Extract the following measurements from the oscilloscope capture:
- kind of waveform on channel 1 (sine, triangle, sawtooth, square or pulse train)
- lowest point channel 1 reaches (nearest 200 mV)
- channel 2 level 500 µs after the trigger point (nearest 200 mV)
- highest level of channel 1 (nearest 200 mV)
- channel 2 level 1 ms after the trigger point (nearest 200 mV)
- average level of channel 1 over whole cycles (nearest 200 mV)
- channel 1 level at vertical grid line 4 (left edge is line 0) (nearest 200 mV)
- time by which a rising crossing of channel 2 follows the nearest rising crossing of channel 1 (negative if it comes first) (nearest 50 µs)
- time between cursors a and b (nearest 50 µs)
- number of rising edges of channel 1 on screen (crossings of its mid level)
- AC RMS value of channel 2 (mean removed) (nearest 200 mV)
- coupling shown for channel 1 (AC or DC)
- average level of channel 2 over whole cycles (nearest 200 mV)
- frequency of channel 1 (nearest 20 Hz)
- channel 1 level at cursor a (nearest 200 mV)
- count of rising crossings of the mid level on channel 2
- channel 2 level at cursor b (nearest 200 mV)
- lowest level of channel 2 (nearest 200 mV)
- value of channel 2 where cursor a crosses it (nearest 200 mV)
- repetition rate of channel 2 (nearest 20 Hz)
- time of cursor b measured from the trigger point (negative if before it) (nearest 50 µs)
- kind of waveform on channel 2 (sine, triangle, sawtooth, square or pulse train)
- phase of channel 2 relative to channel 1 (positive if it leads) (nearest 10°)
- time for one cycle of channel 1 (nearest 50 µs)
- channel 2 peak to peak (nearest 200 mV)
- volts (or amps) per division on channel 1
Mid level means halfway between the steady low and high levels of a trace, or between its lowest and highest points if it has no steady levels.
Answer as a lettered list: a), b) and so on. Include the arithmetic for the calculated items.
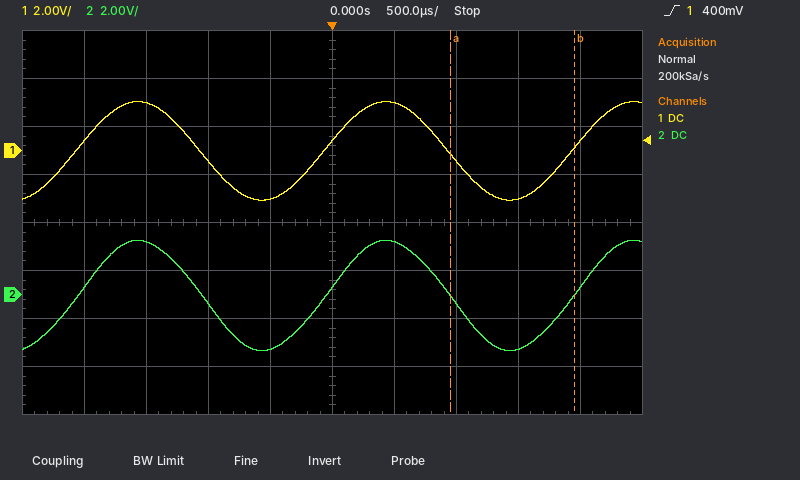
a) sine
b) -2.0 V
c) 2.2 V
d) 2.0 V
e) -400 mV
f) (2.0 V + (-2.0 V)) / 2 ≈ 0.0 V
g) -2.0 V
h) 0 µs
i) 1.00 ms
j) 3
k) 4.6 V / (2√2) ≈ 1.6 V
l) DC
m) (2.2 V + (-2.4 V)) / 2 ≈ 0.0 V
n) 1 / 2.00 ms ≈ 500 Hz
o) -200 mV
p) 3
q) 0.0 V
r) -2.4 V
s) 0.0 V
t) 1 / 2.00 ms ≈ 500 Hz
u) +1.95 ms
v) sine
w) −360° × (0 µs) / 2.00 ms ≈ 0°
x) 2.00 ms
y) 2.2 V − (-2.4 V) = 4.6 V
z) 2 V
